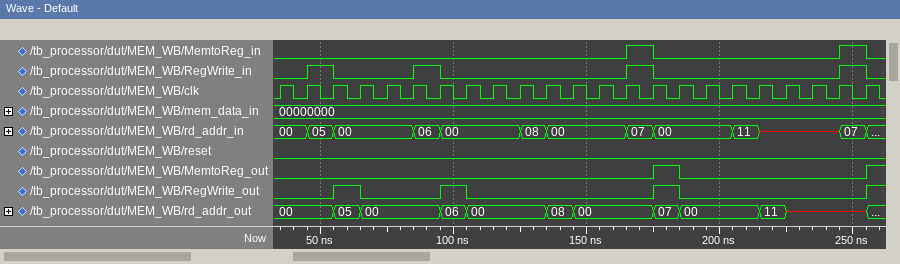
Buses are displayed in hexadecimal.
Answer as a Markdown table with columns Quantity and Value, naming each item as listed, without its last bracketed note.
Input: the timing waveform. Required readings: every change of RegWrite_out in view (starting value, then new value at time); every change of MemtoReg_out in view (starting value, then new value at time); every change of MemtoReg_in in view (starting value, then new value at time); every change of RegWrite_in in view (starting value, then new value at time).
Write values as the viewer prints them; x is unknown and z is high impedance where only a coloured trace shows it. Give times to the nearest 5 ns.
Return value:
| Quantity | Value |
|---|---|
| every change of RegWrite_out in view | 0, 1 at 55 ns, 0 at 65 ns, 1 at 95 ns, 0 at 105 ns, 1 at 175 ns, 0 at 185 ns, 1 at 255 ns |
| every change of MemtoReg_out in view | 0, 1 at 175 ns, 0 at 185 ns, 1 at 255 ns |
| every change of MemtoReg_in in view | 0, 1 at 165 ns, 0 at 175 ns, 1 at 245 ns, 0 at 255 ns |
| every change of RegWrite_in in view | 0, 1 at 45 ns, 0 at 55 ns, 1 at 85 ns, 0 at 95 ns, 1 at 165 ns, 0 at 175 ns, 1 at 245 ns, 0 at 255 ns |
